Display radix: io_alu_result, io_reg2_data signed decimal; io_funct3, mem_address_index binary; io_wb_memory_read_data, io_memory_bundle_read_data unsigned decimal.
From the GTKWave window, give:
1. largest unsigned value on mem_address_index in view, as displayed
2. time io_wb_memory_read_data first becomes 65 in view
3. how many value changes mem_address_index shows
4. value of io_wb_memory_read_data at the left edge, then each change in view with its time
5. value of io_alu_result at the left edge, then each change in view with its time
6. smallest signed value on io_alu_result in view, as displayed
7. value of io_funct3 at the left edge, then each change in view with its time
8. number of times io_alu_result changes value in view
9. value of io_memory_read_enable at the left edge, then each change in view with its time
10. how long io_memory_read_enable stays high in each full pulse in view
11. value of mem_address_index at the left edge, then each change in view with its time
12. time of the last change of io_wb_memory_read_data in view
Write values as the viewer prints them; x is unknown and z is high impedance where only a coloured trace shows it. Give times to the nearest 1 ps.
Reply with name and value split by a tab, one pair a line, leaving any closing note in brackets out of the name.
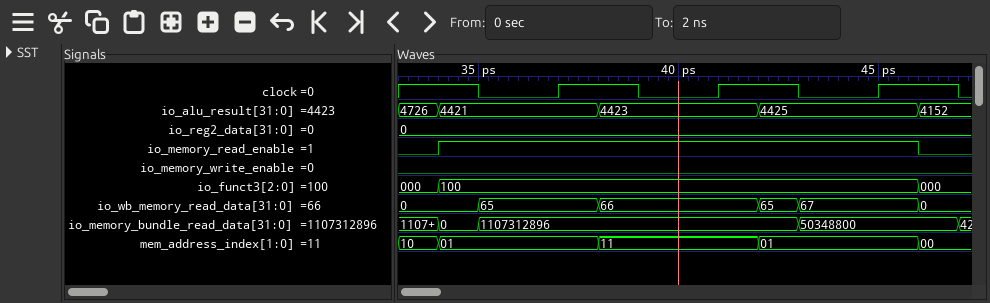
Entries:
largest unsigned value on mem_address_index in view, as displayed	11
time io_wb_memory_read_data first becomes 65 in view	35 ps
how many value changes mem_address_index shows	4
value of io_wb_memory_read_data at the left edge, then each change in view with its time	0, 65 at 35 ps, 66 at 38 ps, 65 at 42 ps, 67 at 43 ps, 0 at 46 ps
value of io_alu_result at the left edge, then each change in view with its time	4726, 4421 at 34 ps, 4423 at 38 ps, 4425 at 42 ps, 4152 at 46 ps
smallest signed value on io_alu_result in view, as displayed	4152
value of io_funct3 at the left edge, then each change in view with its time	000, 100 at 34 ps, 000 at 46 ps
number of times io_alu_result changes value in view	4
value of io_memory_read_enable at the left edge, then each change in view with its time	0, 1 at 34 ps, 0 at 46 ps
how long io_memory_read_enable stays high in each full pulse in view	12 ps
value of mem_address_index at the left edge, then each change in view with its time	10, 01 at 34 ps, 11 at 38 ps, 01 at 42 ps, 00 at 46 ps
time of the last change of io_wb_memory_read_data in view	46 ps
